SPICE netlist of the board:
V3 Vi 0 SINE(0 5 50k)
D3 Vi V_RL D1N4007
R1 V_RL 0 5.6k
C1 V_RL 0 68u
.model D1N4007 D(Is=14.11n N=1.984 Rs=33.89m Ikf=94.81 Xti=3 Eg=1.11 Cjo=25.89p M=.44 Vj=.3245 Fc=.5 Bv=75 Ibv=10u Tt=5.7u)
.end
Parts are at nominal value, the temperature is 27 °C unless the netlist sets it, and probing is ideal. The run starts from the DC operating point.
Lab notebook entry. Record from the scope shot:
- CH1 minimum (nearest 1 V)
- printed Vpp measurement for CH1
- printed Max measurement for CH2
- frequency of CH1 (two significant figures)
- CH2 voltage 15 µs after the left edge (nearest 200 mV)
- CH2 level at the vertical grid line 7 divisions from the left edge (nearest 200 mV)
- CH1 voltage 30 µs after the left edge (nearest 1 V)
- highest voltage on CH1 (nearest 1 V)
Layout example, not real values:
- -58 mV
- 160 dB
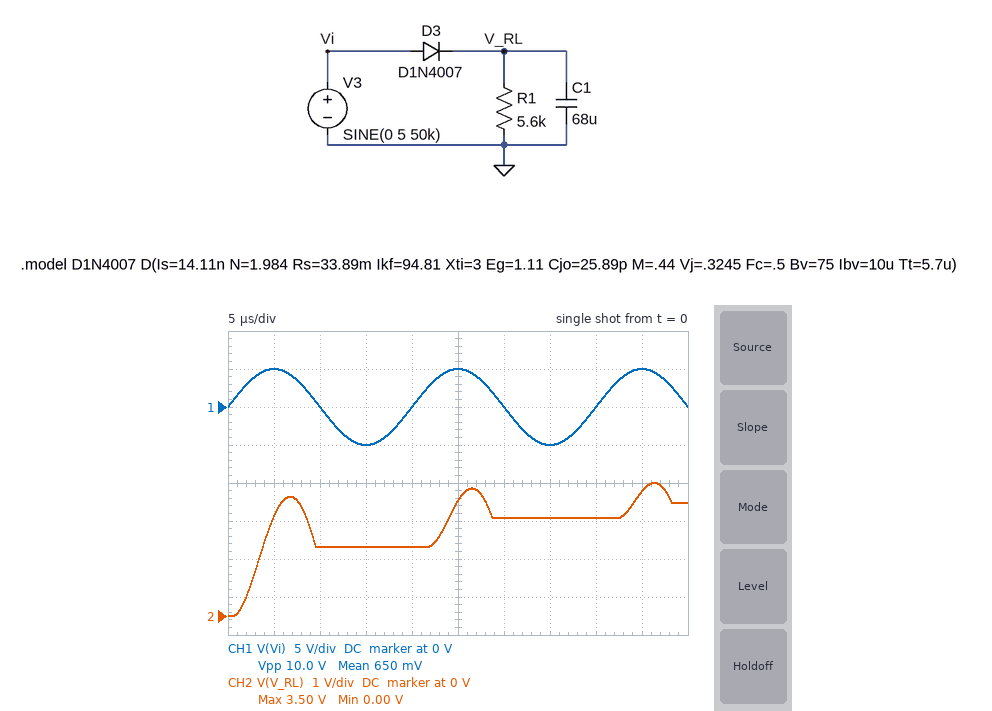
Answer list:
- -5 V
- 10.0 V
- 3.50 V
- 50 kHz
- 1.8 V
- 2.6 V
- 0 V
- 5 V
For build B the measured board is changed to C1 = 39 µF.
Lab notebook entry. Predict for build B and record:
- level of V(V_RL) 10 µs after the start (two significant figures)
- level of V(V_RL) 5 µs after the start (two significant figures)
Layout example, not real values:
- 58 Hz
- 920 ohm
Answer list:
- 2.0 V
- 3.3 V
